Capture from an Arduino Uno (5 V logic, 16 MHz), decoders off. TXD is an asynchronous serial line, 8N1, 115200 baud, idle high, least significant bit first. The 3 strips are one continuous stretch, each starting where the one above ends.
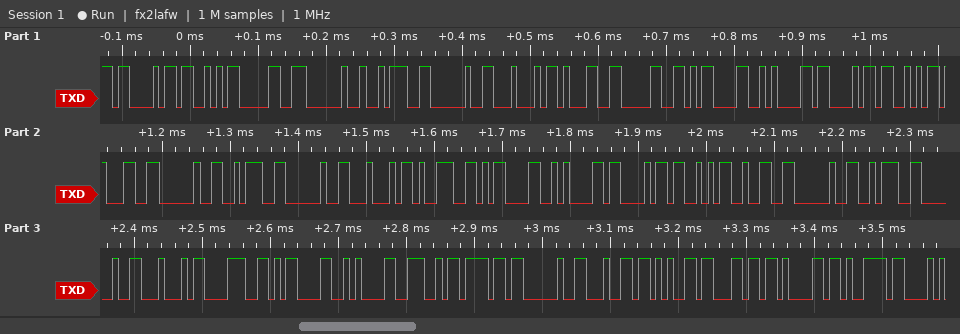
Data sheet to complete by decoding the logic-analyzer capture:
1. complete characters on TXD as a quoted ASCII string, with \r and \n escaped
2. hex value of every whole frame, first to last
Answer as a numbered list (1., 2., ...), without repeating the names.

1. "CS0 : D10\r\nCS1 : D9\r\nCS2 : D8\r\nNo delay"
2. 43 53 30 20 3A 20 44 31 30 0D 0A 43 53 31 20 3A 20 44 39 0D 0A 43 53 32 20 3A 20 44 38 0D 0A 4E 6F 20 64 65 6C 61 79
